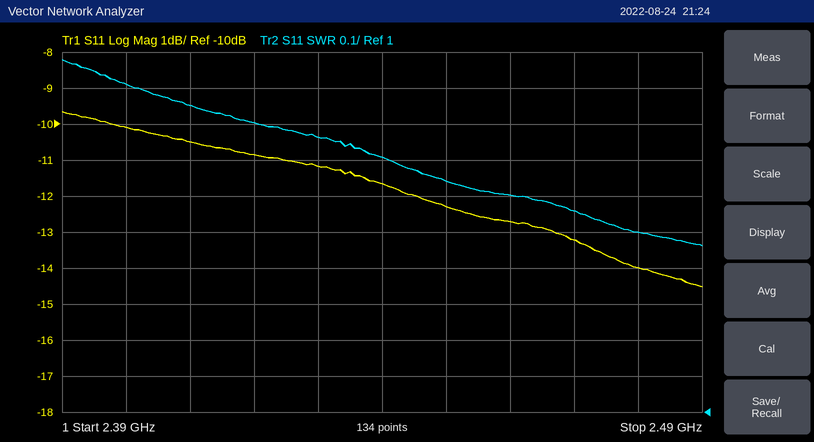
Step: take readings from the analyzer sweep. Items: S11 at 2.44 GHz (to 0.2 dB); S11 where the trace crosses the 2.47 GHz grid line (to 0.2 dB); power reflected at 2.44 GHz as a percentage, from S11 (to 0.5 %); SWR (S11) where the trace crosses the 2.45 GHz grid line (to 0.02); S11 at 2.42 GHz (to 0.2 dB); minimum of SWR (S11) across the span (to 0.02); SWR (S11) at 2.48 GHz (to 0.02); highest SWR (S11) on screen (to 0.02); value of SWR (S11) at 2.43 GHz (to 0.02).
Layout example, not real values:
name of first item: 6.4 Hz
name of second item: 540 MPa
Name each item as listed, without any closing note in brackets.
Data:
S11 at 2.44 GHz: -11.6 dB
S11 where the trace crosses the 2.47 GHz grid line: -13.2 dB
power reflected at 2.44 GHz as a percentage, from S11: 7.0 %
SWR (S11) where the trace crosses the 2.45 GHz grid line: 1.64
S11 at 2.42 GHz: -10.8 dB
minimum of SWR (S11) across the span: 1.46
SWR (S11) at 2.48 GHz: 1.50
highest SWR (S11) on screen: 1.98
value of SWR (S11) at 2.43 GHz: 1.76
